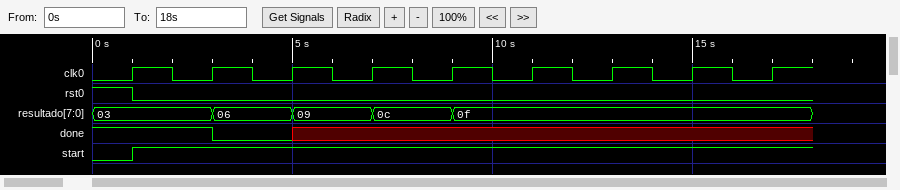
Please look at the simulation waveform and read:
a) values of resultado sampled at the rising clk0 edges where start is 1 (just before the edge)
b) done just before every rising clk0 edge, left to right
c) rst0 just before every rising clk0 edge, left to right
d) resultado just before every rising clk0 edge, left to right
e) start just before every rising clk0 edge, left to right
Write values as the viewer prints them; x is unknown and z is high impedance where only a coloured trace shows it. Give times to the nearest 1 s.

03, 06, 09, 0c, 0f, 0f, 0f, 0f
1 1 0 x x x x x x
1 0 0 0 0 0 0 0 0
03, 03, 06, 09, 0c, 0f, 0f, 0f, 0f
0 1 1 1 1 1 1 1 1
